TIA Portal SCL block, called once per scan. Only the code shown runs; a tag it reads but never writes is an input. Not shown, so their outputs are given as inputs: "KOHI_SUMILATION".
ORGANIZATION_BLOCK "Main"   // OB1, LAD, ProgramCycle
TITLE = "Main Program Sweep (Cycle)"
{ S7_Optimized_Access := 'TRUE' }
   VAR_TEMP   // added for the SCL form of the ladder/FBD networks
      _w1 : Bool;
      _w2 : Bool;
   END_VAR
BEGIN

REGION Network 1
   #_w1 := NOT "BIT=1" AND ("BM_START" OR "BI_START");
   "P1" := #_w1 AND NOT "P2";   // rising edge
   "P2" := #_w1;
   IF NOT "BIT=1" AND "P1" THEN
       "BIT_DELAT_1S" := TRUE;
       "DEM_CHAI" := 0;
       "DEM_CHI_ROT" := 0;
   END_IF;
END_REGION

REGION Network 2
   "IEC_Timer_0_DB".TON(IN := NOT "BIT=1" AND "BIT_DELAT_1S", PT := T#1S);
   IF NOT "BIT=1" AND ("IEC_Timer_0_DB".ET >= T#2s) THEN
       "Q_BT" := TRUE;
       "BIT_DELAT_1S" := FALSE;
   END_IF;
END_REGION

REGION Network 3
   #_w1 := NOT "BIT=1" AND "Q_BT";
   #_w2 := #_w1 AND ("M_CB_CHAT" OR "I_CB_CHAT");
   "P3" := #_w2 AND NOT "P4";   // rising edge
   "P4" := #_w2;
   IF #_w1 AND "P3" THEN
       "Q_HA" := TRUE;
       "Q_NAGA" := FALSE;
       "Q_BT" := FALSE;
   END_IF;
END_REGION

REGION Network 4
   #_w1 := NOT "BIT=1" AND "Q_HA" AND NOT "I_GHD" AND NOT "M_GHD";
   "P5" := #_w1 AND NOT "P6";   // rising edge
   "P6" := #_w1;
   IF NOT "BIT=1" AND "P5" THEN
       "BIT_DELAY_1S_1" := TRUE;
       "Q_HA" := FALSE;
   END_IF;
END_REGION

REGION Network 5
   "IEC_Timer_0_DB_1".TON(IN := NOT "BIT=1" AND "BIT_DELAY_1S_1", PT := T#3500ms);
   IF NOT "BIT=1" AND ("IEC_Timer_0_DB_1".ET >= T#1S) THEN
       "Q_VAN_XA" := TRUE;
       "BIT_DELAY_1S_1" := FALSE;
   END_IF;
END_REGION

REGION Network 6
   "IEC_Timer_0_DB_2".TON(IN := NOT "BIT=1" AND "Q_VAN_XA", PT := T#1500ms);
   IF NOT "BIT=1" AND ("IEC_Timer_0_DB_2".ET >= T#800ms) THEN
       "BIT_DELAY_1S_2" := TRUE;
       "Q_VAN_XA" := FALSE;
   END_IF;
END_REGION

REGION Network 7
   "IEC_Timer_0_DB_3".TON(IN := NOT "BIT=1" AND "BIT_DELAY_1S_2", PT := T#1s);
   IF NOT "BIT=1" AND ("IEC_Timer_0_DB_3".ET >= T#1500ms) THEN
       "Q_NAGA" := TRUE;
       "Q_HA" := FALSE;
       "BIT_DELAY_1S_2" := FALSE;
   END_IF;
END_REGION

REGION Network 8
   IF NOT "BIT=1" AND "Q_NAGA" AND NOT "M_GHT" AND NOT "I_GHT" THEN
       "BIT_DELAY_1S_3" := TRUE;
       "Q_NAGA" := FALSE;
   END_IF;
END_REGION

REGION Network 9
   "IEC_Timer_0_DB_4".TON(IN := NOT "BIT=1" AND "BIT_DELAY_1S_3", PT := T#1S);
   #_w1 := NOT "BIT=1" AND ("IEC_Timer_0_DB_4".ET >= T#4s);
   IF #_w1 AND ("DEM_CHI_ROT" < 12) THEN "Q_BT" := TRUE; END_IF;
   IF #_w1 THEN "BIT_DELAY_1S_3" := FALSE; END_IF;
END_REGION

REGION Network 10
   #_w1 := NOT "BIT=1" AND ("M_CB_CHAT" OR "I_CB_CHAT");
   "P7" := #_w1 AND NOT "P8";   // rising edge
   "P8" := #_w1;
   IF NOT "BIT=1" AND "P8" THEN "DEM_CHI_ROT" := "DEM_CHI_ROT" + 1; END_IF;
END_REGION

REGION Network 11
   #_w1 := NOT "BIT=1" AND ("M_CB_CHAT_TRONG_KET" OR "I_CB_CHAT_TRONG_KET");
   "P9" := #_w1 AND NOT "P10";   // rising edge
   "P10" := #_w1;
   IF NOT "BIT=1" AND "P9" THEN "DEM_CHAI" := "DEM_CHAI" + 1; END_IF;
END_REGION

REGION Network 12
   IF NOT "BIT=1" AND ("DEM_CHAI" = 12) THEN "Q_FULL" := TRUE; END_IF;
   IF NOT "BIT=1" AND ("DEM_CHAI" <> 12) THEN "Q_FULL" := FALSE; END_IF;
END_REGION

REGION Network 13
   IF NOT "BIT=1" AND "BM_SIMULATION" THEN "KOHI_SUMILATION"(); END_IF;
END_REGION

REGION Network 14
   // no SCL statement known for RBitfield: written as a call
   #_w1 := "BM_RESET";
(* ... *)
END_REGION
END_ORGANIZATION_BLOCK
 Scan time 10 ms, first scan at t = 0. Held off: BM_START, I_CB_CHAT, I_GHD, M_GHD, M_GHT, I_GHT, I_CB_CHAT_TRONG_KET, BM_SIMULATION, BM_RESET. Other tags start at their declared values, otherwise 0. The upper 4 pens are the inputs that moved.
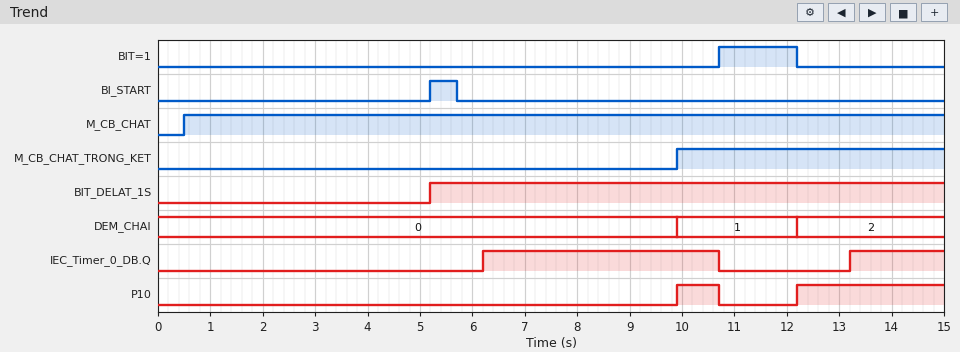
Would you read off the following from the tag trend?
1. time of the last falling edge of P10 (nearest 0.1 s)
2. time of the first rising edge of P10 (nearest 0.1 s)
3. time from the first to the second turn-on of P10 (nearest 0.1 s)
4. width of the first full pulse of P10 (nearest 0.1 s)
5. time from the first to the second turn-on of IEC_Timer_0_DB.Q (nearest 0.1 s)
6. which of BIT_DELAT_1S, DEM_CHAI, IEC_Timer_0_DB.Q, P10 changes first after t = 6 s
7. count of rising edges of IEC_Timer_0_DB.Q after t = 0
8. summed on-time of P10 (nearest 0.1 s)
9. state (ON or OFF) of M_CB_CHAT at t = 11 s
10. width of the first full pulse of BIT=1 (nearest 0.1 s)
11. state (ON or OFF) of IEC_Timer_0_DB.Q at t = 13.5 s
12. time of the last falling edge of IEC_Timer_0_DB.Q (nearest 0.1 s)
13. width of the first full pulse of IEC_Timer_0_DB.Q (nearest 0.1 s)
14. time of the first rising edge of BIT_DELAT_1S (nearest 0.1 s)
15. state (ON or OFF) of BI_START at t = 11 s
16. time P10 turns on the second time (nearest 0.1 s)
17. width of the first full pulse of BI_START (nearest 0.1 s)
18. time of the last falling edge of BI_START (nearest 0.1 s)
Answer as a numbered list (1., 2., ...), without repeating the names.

1. 10.7 s
2. 9.9 s
3. 2.3 s
4. 0.8 s
5. 7.0 s
6. IEC_Timer_0_DB.Q
7. 2
8. 3.6 s
9. ON
10. 1.5 s
11. ON
12. 10.7 s
13. 4.5 s
14. 5.2 s
15. OFF
16. 12.2 s
17. 0.5 s
18. 5.7 s
